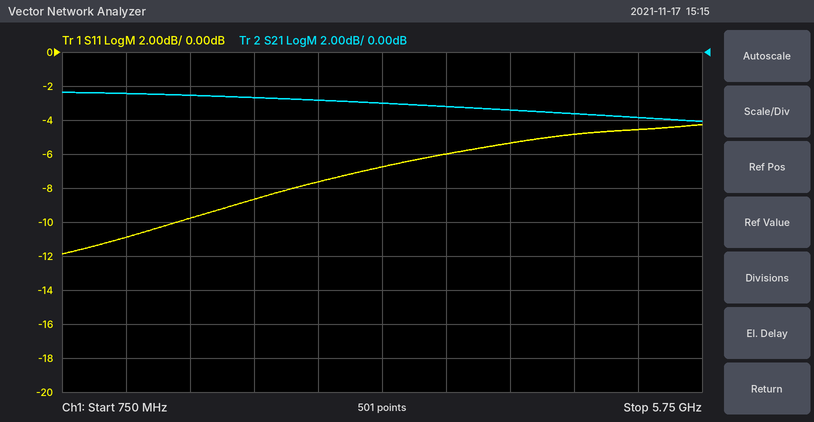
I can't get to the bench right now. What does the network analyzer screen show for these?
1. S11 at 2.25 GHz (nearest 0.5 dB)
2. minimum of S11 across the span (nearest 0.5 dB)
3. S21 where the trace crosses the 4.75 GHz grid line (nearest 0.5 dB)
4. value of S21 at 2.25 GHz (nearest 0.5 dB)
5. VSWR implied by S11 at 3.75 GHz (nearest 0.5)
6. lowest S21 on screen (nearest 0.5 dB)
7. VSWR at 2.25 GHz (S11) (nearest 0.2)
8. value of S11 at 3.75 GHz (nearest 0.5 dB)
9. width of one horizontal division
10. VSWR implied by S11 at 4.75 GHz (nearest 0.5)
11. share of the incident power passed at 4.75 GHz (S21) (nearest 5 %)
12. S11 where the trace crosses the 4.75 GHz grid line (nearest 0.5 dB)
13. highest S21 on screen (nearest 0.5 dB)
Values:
-8.5 dB
-12.0 dB
-3.5 dB
-2.5 dB
3.0
-4.0 dB
2.2
-6.0 dB
500 MHz
3.5
45 %
-5.0 dB
-2.5 dB
